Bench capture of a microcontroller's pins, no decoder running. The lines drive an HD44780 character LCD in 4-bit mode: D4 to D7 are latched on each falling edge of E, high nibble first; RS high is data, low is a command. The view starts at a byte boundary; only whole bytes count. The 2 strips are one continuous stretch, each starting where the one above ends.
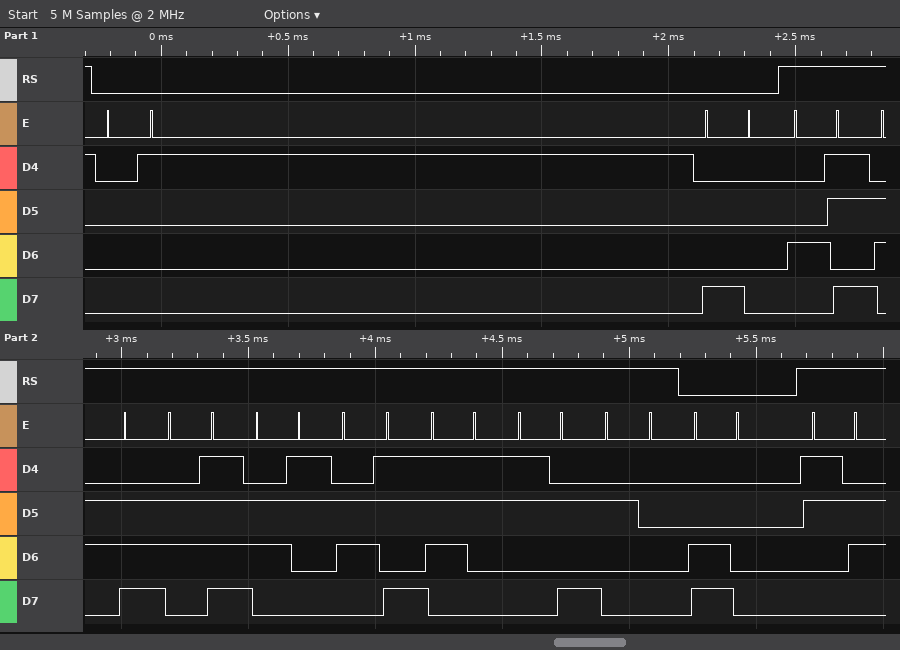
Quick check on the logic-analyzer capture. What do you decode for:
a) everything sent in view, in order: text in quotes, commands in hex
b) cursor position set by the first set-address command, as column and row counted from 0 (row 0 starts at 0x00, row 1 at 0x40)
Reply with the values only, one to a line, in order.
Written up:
0x01 0x80 "Knocks: " 0xC0 "6"
column 0, row 0
